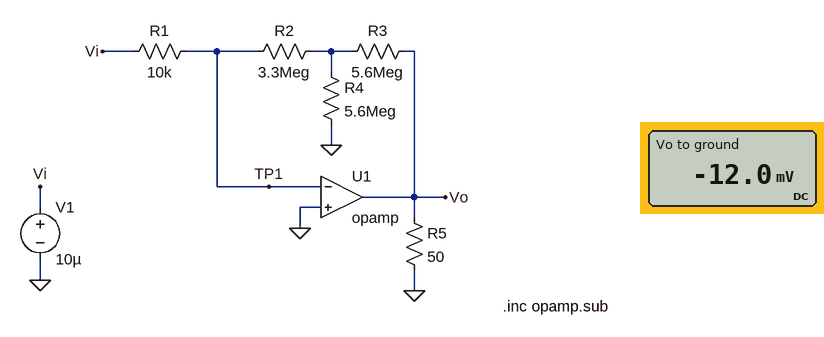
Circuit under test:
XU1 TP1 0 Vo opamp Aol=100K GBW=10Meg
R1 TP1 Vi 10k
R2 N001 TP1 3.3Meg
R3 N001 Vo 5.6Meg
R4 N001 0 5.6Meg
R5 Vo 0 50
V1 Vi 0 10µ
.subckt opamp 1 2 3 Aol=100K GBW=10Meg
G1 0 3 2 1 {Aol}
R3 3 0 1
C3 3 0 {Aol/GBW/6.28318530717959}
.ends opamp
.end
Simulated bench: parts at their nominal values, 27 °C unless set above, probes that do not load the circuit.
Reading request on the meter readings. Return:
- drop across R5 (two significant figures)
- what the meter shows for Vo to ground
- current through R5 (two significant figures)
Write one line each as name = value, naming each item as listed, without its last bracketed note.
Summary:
drop across R5 = 12 mV
what the meter shows for Vo to ground = -12.0 mV
current through R5 = 240 µA
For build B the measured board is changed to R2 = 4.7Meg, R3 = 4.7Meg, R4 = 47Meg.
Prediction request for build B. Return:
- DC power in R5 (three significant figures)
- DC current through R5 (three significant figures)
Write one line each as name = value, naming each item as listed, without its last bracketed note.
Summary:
DC power in R5 = 1.91 µW
DC current through R5 = 195 µA
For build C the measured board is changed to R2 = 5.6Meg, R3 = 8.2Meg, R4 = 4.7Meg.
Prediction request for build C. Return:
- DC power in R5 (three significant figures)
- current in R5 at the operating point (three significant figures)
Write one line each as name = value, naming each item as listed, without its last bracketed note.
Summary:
DC power in R5 = 10.6 µW
current in R5 at the operating point = 460 µA
